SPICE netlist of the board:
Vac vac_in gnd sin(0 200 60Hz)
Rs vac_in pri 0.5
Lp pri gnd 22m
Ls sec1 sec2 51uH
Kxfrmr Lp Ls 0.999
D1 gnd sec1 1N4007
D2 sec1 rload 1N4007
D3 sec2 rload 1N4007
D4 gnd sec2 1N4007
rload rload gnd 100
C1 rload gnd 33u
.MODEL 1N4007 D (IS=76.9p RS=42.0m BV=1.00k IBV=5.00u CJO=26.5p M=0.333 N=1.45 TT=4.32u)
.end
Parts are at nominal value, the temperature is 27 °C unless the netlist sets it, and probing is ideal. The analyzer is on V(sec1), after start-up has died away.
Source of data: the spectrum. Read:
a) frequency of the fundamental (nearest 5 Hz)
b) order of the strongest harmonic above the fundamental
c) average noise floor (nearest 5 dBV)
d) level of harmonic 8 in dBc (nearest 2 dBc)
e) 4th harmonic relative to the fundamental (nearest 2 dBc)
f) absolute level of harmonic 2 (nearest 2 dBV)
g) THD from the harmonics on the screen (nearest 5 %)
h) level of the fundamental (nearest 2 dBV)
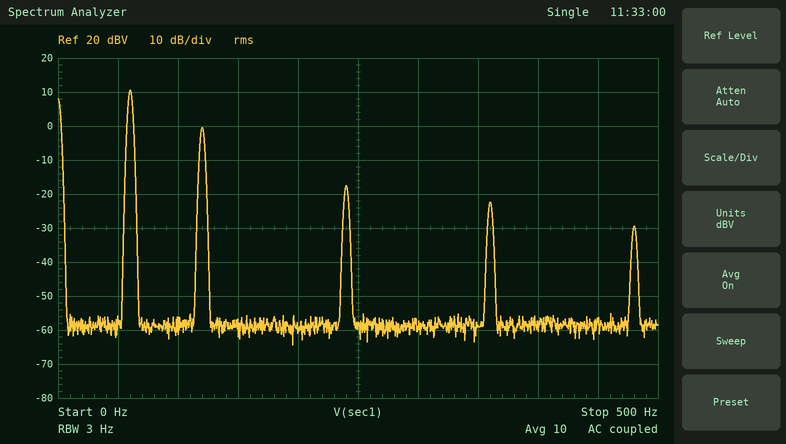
60 Hz
2
-60 dBV
-40 dBc
-28 dBc
0 dBV
30 %
10 dBV
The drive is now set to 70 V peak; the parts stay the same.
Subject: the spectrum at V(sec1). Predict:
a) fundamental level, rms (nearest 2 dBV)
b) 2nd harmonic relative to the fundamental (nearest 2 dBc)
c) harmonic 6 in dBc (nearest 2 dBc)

2 dBV
-14 dBc
-36 dBc
